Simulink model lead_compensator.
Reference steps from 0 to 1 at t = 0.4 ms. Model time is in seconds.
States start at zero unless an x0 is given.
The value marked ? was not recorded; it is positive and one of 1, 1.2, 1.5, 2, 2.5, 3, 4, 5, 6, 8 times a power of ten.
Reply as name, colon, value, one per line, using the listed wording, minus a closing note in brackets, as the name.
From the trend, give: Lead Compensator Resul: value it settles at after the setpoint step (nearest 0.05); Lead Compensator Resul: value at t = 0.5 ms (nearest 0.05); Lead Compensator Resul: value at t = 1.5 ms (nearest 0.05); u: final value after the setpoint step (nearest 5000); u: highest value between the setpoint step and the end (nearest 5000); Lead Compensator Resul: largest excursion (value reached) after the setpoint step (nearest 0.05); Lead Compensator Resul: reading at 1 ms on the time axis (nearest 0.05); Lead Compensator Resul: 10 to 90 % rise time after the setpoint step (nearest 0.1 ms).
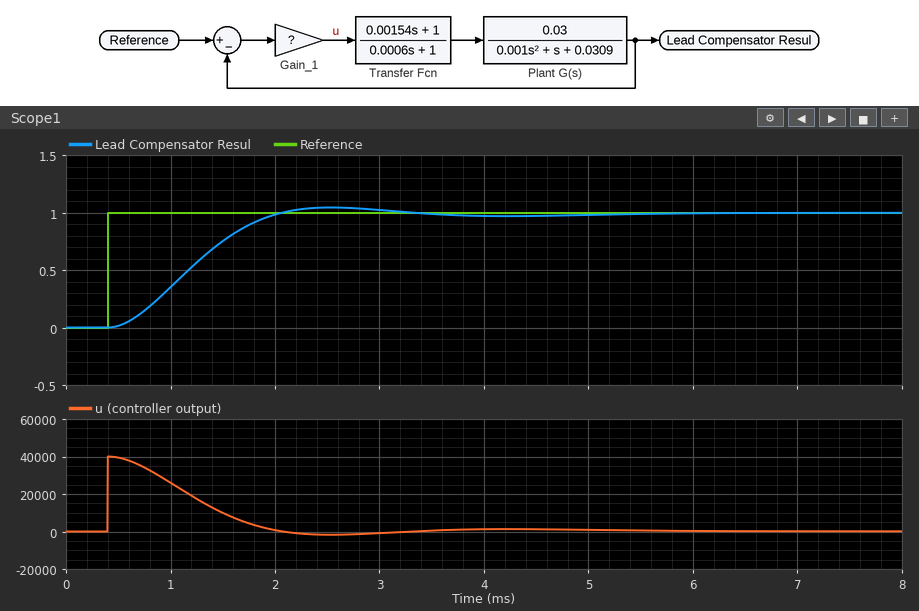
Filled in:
Lead Compensator Resul: value it settles at after the setpoint step: 1.00
Lead Compensator Resul: value at t = 0.5 ms: 0.00
Lead Compensator Resul: value at t = 1.5 ms: 0.75
u: final value after the setpoint step: 0
u: highest value between the setpoint step and the end: 40000
Lead Compensator Resul: largest excursion (value reached) after the setpoint step: 1.05
Lead Compensator Resul: reading at 1 ms on the time axis: 0.35
Lead Compensator Resul: 10 to 90 % rise time after the setpoint step: 1.1 ms
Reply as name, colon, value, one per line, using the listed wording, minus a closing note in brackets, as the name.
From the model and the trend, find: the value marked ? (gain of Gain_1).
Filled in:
the value marked ?: 40000
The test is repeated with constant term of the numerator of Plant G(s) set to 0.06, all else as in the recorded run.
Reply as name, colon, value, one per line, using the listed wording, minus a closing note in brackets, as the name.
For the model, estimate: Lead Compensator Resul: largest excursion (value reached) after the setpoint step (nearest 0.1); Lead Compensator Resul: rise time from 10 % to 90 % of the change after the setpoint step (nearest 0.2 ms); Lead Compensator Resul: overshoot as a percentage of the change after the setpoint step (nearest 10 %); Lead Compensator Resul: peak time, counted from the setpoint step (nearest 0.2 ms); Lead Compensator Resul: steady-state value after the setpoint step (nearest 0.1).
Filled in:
Lead Compensator Resul: largest excursion (value reached) after the setpoint step: 1.2
Lead Compensator Resul: rise time from 10 % to 90 % of the change after the setpoint step: 0.6 ms
Lead Compensator Resul: overshoot as a percentage of the change after the setpoint step: 20 %
Lead Compensator Resul: peak time, counted from the setpoint step: 1.4 ms
Lead Compensator Resul: steady-state value after the setpoint step: 1.0
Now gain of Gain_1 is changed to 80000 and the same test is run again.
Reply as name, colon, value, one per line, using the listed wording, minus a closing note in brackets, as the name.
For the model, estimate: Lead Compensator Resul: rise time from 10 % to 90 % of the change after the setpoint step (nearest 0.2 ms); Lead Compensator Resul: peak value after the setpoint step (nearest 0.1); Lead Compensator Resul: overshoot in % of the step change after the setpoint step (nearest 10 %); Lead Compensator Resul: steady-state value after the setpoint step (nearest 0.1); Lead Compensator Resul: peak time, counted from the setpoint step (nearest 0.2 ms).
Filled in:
Lead Compensator Resul: rise time from 10 % to 90 % of the change after the setpoint step: 0.6 ms
Lead Compensator Resul: peak value after the setpoint step: 1.2
Lead Compensator Resul: overshoot in % of the step change after the setpoint step: 20 %
Lead Compensator Resul: steady-state value after the setpoint step: 1.0
Lead Compensator Resul: peak time, counted from the setpoint step: 1.4 ms
